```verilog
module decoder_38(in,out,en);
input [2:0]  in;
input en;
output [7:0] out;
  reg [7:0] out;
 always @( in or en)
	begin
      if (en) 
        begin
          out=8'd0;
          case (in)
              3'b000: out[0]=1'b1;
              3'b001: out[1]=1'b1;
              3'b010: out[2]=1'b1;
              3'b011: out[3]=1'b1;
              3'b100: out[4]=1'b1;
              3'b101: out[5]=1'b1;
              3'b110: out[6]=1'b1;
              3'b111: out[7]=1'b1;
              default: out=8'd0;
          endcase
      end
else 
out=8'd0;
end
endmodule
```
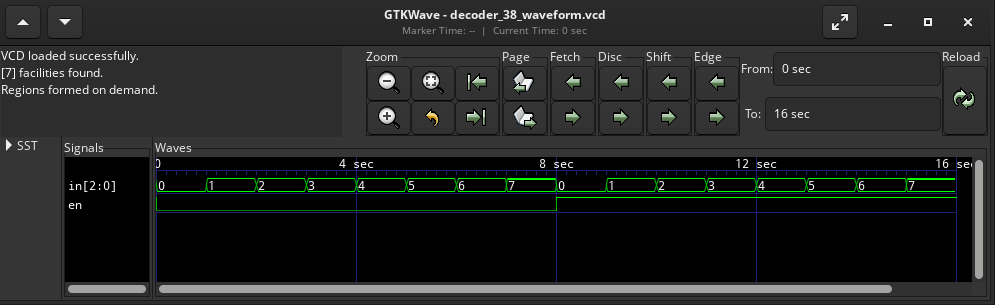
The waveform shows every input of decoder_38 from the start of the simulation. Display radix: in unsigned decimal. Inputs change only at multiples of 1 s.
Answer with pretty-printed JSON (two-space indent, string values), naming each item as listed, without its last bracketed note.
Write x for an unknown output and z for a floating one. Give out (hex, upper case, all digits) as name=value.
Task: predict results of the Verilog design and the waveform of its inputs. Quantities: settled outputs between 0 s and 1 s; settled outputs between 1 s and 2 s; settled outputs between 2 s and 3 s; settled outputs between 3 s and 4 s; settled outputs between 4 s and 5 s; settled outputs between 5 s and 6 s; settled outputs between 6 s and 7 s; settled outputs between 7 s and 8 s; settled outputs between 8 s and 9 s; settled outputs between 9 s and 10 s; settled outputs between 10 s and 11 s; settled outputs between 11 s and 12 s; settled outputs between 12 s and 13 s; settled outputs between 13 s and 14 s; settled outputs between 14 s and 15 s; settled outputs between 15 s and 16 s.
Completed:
{
  "settled outputs between 0 s and 1 s": "out=00",
  "settled outputs between 1 s and 2 s": "out=00",
  "settled outputs between 2 s and 3 s": "out=00",
  "settled outputs between 3 s and 4 s": "out=00",
  "settled outputs between 4 s and 5 s": "out=00",
  "settled outputs between 5 s and 6 s": "out=00",
  "settled outputs between 6 s and 7 s": "out=00",
  "settled outputs between 7 s and 8 s": "out=00",
  "settled outputs between 8 s and 9 s": "out=01",
  "settled outputs between 9 s and 10 s": "out=02",
  "settled outputs between 10 s and 11 s": "out=04",
  "settled outputs between 11 s and 12 s": "out=08",
  "settled outputs between 12 s and 13 s": "out=10",
  "settled outputs between 13 s and 14 s": "out=20",
  "settled outputs between 14 s and 15 s": "out=40",
  "settled outputs between 15 s and 16 s": "out=80"
}
